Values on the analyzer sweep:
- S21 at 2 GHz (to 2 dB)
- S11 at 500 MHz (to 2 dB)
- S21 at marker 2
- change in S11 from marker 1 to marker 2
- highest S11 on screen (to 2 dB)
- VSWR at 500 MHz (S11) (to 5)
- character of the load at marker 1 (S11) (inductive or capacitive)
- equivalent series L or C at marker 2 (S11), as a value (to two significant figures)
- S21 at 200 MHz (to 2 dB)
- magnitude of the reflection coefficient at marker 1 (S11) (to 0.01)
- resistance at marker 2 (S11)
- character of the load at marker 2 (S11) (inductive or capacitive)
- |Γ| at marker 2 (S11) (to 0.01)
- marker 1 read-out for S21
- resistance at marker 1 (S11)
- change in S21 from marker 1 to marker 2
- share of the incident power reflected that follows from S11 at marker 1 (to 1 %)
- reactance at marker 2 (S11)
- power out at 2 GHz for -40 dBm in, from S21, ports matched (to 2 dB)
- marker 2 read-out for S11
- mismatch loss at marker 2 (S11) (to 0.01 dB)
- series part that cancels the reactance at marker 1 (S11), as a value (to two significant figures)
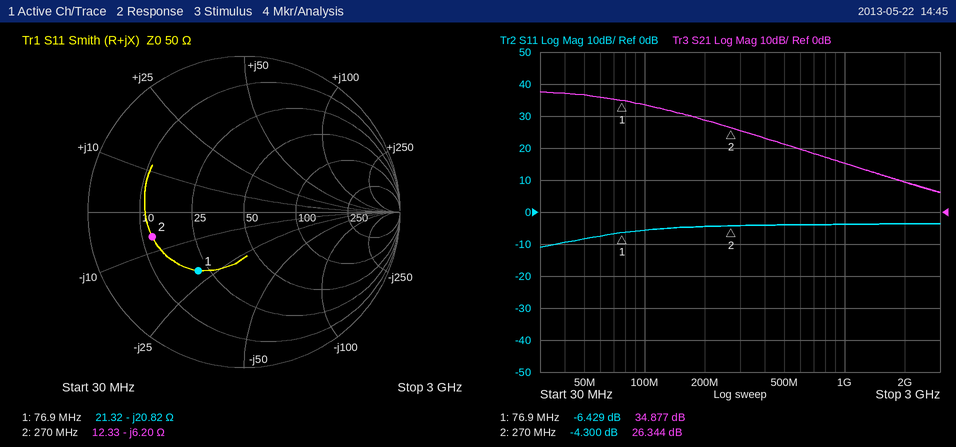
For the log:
10 dB
-4 dB
26.344 dB
2.129 dB
-4 dB
5
capacitive
95 pF
28 dB
0.48
12.33 Ω
capacitive
0.61
34.877 dB
21.32 Ω
-8.533 dB
23 %
-6.20 Ω
-30 dBm
-4.300 dB
2.02 dB
43 nH
